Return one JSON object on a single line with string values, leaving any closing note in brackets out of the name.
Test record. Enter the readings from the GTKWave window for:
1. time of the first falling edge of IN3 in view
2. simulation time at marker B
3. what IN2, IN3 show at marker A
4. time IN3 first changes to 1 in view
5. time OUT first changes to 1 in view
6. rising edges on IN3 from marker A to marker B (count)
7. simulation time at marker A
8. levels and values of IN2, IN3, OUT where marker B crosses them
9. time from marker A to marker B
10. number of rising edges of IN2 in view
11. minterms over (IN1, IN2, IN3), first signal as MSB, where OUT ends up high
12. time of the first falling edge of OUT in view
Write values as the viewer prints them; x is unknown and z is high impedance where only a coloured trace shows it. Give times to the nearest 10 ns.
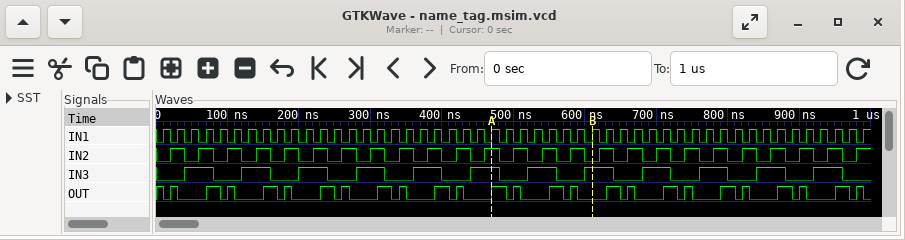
{"time of the first falling edge of IN3 in view": "80 ns", "simulation time at marker B": "610 ns", "what IN2, IN3 show at marker A": "IN2=1, IN3=1", "time IN3 first changes to 1 in view": "40 ns", "time OUT first changes to 1 in view": "20 ns", "rising edges on IN3 from marker A to marker B": "2", "simulation time at marker A": "470 ns", "levels and values of IN2, IN3, OUT where marker B crosses them": "IN2=0, IN3=1, OUT=0", "time from marker A to marker B": "140 ns", "number of rising edges of IN2 in view": "25", "minterms over (IN1, IN2, IN3), first signal as MSB, where OUT ends up high": "0, 2, 7", "time of the first falling edge of OUT in view": "10 ns"}
